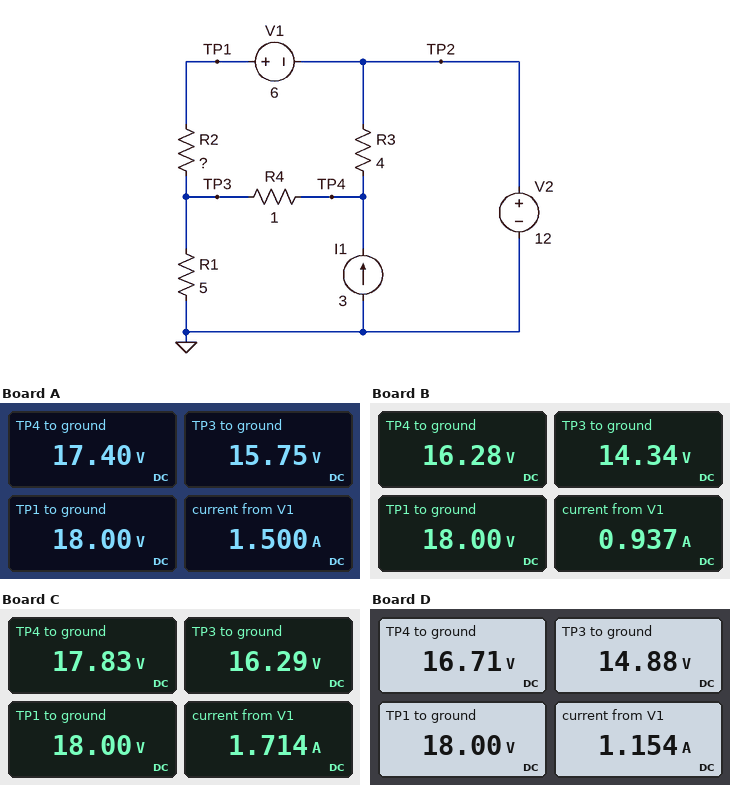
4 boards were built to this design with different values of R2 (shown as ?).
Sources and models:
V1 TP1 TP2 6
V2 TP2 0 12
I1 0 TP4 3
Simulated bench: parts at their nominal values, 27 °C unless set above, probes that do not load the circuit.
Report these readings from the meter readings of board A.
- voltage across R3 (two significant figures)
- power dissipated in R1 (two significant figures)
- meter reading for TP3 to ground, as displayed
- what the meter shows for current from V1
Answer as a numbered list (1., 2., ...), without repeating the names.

1. 5.4 V
2. 50 W
3. 15.75 V
4. 1.500 A
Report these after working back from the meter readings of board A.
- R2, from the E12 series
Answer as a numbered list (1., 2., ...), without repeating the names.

1. 1.5 Ω
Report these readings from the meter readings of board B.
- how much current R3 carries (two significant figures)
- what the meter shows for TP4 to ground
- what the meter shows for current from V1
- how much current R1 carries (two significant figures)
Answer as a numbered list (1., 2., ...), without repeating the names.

1. 1.1 A
2. 16.28 V
3. 0.937 A
4. 2.9 A
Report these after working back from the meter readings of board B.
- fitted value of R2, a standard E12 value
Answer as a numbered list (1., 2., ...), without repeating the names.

1. 3.9 Ω
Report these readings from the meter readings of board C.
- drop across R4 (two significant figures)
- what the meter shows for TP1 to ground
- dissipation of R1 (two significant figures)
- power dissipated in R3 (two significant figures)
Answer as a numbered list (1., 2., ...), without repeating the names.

1. 1.5 V
2. 18.00 V
3. 53 W
4. 8.5 W
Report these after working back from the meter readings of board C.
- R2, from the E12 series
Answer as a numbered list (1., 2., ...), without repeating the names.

1. 1 Ω
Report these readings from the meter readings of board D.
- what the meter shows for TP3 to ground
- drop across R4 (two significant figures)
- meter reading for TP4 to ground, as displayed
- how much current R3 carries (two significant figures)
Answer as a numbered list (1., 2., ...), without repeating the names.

1. 14.88 V
2. 1.8 V
3. 16.71 V
4. 1.2 A
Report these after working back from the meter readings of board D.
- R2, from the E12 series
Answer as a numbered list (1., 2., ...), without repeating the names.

1. 2.7 Ω
